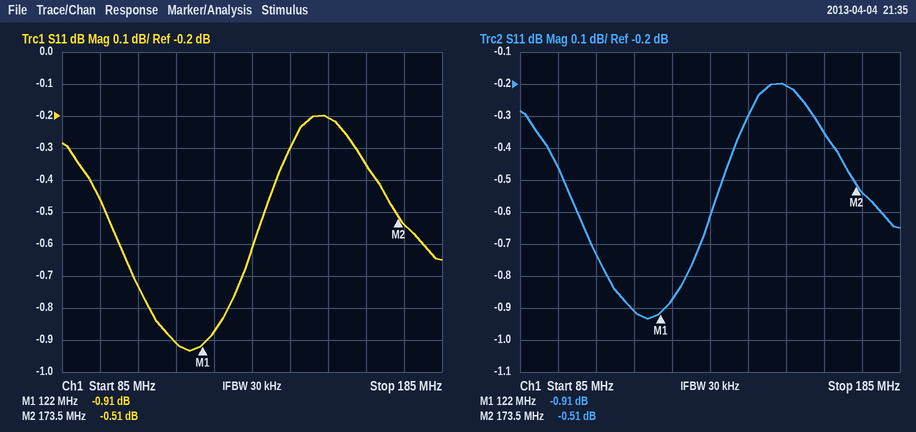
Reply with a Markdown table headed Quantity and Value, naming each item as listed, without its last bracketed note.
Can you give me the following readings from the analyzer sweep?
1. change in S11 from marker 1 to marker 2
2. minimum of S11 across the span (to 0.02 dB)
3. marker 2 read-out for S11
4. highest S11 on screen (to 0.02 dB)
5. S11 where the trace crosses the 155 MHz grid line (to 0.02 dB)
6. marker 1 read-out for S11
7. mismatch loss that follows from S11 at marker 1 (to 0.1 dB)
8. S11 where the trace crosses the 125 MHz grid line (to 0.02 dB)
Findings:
| Quantity | Value |
|---|---|
| change in S11 from marker 1 to marker 2 | 0.40 dB |
| minimum of S11 across the span | -0.94 dB |
| marker 2 read-out for S11 | -0.51 dB |
| highest S11 on screen | -0.20 dB |
| S11 where the trace crosses the 155 MHz grid line | -0.20 dB |
| marker 1 read-out for S11 | -0.91 dB |
| mismatch loss that follows from S11 at marker 1 | 7.2 dB |
| S11 where the trace crosses the 125 MHz grid line | -0.88 dB |
